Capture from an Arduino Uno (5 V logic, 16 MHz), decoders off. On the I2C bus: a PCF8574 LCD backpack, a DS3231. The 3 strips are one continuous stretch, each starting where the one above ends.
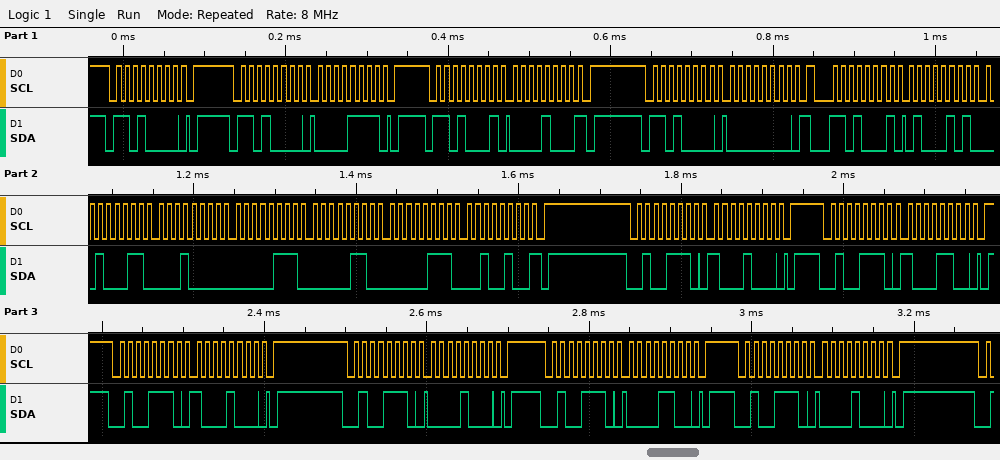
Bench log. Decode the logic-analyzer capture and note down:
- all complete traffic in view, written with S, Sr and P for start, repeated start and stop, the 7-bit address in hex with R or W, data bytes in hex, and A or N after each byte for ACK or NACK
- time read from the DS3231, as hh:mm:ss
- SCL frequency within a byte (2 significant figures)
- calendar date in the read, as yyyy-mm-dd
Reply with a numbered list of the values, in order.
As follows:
1. S 68W A P S 68W A 0F A P S 68R A 08 N P S 68W A 00 A Sr 68R A 45 A 23 A 10 A 07 A 06 A 07 A 24 N P S 27W A 88 A P S 27W A 8C A P S 27W A 88 A P S 27W A 08 A P S 27W A 0C A P S 27W A 08 A P
2. 10:23:45
3. 100 kHz
4. 2024-07-06
